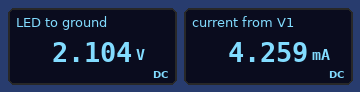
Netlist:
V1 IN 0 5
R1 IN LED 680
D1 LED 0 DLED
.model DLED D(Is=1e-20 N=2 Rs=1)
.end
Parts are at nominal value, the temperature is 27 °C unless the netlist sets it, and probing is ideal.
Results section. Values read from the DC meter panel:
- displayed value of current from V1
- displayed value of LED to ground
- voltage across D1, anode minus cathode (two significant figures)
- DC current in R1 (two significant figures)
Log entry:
4.259 mA
2.104 V
2.1 V
4.3 mA
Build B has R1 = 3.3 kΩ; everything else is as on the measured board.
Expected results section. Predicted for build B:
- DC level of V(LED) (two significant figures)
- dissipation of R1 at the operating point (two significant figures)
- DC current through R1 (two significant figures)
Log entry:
2.0 V
2.7 mW
900 µA
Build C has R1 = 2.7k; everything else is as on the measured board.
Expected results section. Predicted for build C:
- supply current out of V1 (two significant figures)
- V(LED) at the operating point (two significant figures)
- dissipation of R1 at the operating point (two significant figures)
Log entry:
1.1 mA
2.0 V
3.3 mW
